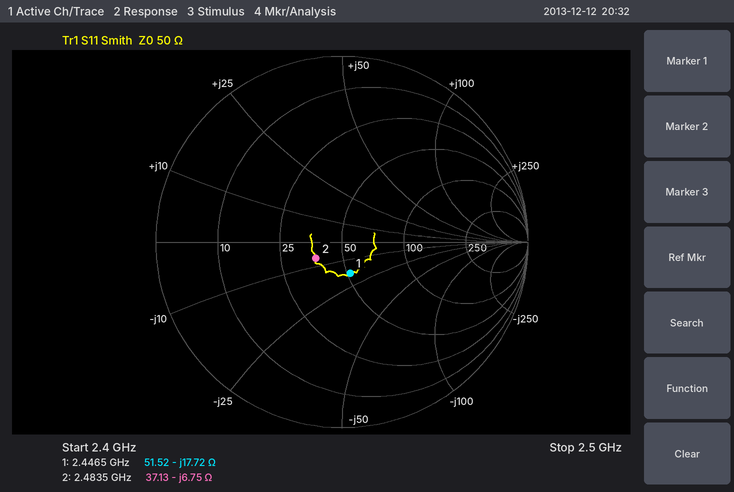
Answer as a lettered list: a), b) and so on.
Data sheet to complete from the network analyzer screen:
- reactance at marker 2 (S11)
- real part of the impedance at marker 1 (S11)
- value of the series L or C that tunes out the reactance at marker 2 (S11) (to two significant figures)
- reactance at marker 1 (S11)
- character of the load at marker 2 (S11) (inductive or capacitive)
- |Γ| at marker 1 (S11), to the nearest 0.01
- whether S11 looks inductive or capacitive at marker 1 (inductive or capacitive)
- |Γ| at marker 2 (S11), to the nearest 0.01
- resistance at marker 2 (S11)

a) -6.75 Ω
b) 51.52 Ω
c) 430 pH
d) -17.72 Ω
e) capacitive
f) 0.17
g) capacitive
h) 0.17
i) 37.13 Ω
